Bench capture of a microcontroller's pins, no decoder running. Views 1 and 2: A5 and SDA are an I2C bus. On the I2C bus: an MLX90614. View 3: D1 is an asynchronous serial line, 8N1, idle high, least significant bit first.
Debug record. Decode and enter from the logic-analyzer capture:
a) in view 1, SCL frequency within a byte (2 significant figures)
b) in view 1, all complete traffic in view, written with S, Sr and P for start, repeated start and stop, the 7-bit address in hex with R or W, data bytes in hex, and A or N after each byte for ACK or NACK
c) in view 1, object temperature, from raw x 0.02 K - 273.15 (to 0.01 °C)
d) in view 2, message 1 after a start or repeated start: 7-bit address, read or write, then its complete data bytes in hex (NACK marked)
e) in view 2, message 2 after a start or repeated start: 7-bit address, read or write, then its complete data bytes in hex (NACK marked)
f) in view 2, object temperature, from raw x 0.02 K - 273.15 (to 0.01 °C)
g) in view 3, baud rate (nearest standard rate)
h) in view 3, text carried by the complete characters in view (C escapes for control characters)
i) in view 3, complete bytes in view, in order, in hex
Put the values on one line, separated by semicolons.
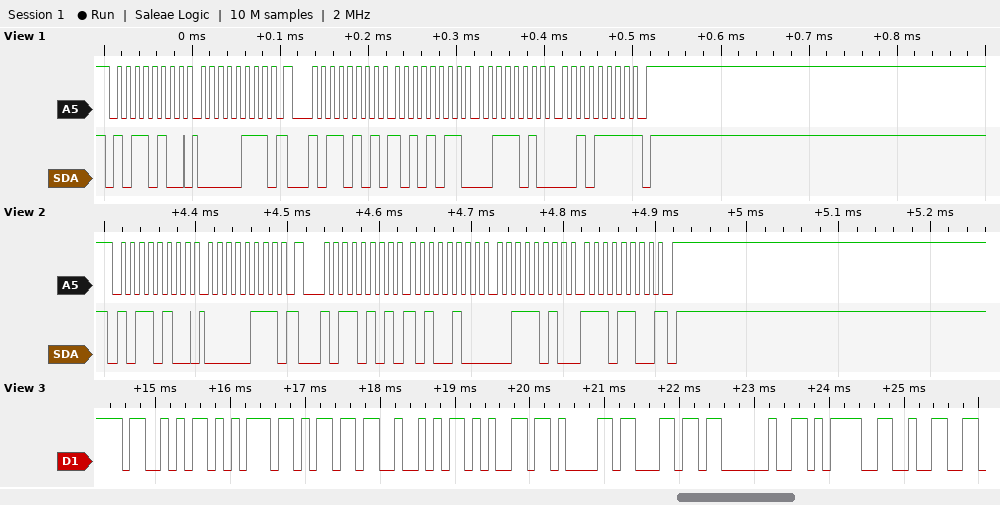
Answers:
100 kHz; S 5AW A 07 A Sr 5AR A AB A 3A A 2F N P; 27.23 °C; 0x5A write: 07; 0x5A read: A4 3A EC NACK; 27.09 °C; 9600 baud; "SumReal =2"; 53 75 6D 52 65 61 6C 20 3D 32
